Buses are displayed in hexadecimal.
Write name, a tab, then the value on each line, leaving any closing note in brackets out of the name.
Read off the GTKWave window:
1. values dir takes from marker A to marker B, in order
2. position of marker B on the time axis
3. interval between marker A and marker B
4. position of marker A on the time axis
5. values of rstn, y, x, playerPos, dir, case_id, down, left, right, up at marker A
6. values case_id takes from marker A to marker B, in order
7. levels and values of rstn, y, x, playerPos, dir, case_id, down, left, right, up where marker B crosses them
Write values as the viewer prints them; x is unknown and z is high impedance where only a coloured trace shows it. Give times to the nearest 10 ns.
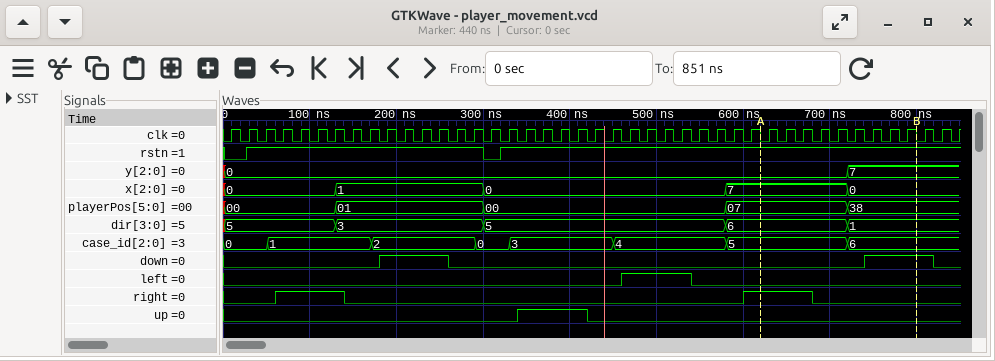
values dir takes from marker A to marker B, in order	6, 1
position of marker B on the time axis	800 ns
interval between marker A and marker B	180 ns
position of marker A on the time axis	620 ns
values of rstn, y, x, playerPos, dir, case_id, down, left, right, up at marker A	rstn=1, y=0, x=7, playerPos=07, dir=6, case_id=5, down=0, left=0, right=1, up=0
values case_id takes from marker A to marker B, in order	5, 6
levels and values of rstn, y, x, playerPos, dir, case_id, down, left, right, up where marker B crosses them	rstn=1, y=7, x=0, playerPos=38, dir=1, case_id=6, down=1, left=0, right=0, up=0
